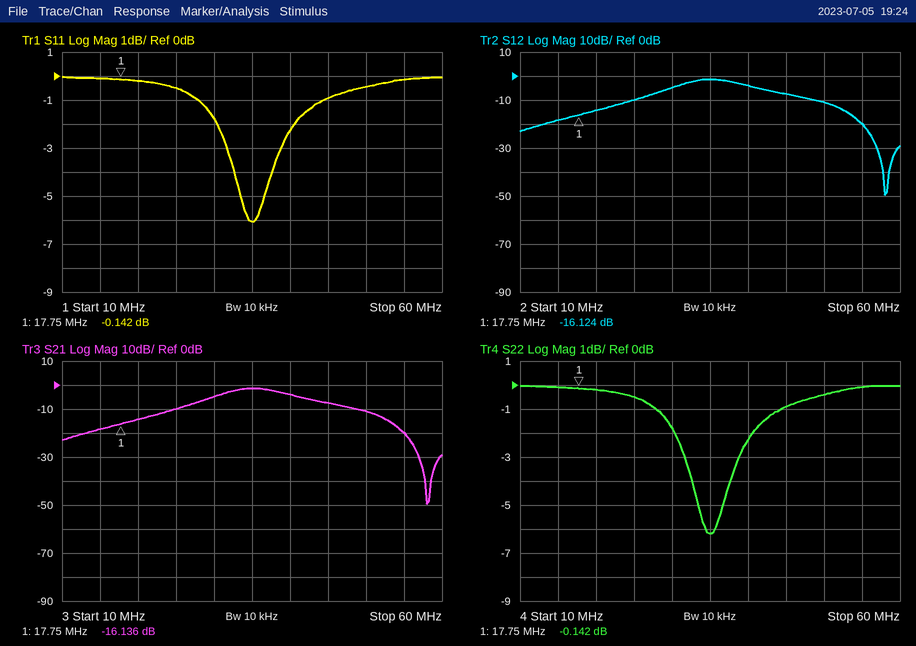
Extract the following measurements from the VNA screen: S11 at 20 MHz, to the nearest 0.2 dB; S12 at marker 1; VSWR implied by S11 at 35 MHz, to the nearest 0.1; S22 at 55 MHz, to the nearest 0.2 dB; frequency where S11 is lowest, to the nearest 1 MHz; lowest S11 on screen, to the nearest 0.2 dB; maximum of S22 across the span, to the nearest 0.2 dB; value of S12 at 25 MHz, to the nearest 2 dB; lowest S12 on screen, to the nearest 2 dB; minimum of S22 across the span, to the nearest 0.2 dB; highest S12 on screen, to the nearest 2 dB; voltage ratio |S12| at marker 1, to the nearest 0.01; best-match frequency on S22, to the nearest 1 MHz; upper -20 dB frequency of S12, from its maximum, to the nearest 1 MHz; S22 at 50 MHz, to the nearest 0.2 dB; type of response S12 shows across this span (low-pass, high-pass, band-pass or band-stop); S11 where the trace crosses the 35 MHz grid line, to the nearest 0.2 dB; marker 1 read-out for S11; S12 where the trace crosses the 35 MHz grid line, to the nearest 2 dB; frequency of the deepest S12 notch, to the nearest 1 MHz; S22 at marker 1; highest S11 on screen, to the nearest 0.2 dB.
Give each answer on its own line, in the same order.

-0.2 dB
-16.124 dB
3.0
0.0 dB
35 MHz
-6.0 dB
0.0 dB
-10 dB
-50 dB
-6.2 dB
-2 dB
0.16
35 MHz
55 MHz
-0.4 dB
band-pass
-6.0 dB
-0.142 dB
-2 dB
58 MHz
-0.142 dB
0.0 dB
